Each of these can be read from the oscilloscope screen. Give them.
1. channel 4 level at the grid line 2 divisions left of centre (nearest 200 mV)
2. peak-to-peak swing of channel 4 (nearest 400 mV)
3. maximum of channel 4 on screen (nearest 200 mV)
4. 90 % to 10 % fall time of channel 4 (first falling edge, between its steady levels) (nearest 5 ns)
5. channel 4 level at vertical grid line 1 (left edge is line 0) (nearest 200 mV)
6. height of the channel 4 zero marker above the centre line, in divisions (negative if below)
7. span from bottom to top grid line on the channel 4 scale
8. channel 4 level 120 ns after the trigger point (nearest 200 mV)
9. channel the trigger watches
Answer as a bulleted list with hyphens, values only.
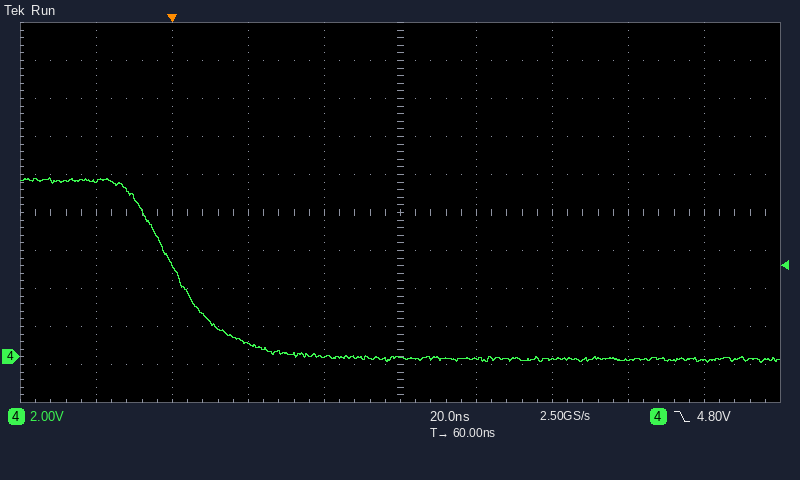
- 600 mV
- 9.6 V
- 9.4 V
- 30 ns
- 9.2 V
- -3.8 div
- 20 V
- -200 mV
- channel 4
